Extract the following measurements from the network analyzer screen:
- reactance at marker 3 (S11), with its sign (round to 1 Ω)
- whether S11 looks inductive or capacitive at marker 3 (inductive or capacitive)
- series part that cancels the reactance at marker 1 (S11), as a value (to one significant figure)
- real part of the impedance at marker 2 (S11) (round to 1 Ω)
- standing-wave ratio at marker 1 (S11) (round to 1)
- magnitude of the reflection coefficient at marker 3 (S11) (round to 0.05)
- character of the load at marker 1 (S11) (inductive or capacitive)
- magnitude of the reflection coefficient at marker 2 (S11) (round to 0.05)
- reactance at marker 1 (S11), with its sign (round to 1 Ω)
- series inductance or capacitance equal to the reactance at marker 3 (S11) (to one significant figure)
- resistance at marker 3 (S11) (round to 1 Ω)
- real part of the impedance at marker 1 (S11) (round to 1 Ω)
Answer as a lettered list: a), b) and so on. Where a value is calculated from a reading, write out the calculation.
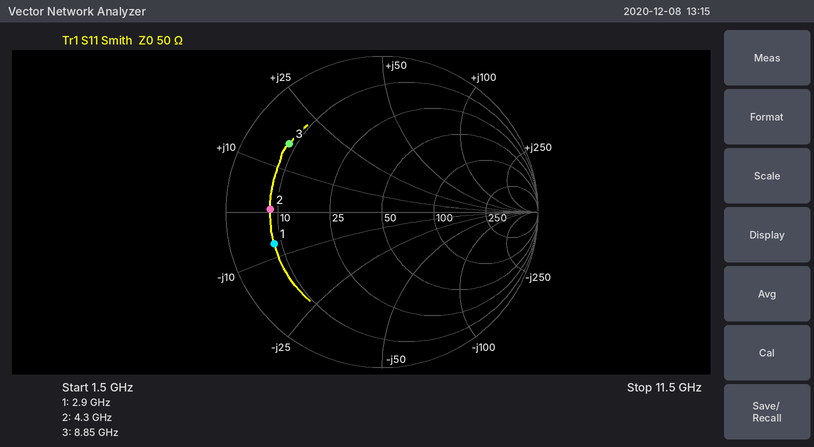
a) +16 Ω
b) inductive
c) L = 7 Ω/(2π × 2.9 GHz) ≈ 384 pH, so 400 pH to one significant figure
d) 8 Ω
e) 6
f) 0.75
g) capacitive
h) 0.70
i) -7 Ω
j) L = 16 Ω/(2π × 8.85 GHz) ≈ 288 pH, so 300 pH to one significant figure
k) 8 Ω
l) 8 Ω
